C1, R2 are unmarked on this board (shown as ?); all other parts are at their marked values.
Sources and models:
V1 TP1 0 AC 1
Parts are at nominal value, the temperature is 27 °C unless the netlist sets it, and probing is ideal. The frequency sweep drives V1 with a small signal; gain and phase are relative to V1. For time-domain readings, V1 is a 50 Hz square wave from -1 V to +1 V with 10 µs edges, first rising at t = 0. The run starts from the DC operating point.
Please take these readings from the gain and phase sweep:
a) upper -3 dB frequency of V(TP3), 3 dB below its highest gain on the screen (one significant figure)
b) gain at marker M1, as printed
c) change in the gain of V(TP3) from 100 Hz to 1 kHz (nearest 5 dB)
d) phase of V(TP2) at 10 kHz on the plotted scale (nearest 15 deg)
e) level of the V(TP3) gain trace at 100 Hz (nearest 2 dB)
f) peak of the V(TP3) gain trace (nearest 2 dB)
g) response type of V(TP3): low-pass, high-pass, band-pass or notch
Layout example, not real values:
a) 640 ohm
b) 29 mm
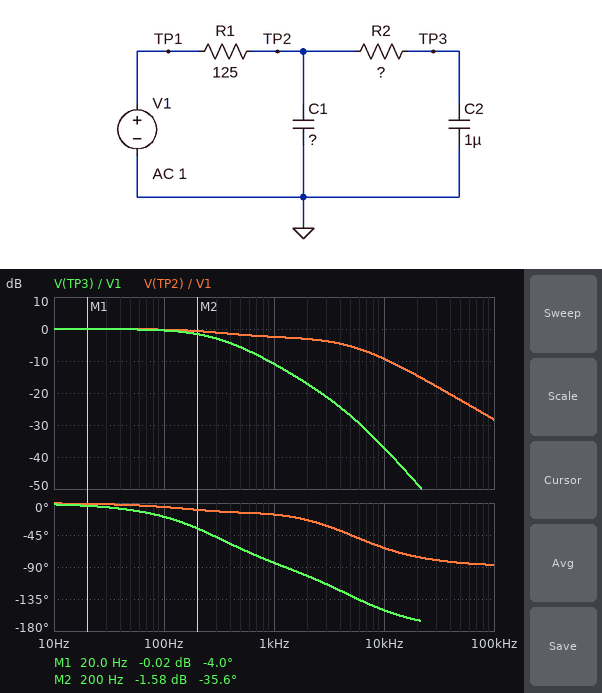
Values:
a) 300 Hz
b) -0.02 dB
c) -10 dB
d) -60 deg
e) 0 dB
f) 0 dB
g) low-pass
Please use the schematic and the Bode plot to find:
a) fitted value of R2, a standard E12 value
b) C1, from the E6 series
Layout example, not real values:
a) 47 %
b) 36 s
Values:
a) 390 Ω
b) 330 nF
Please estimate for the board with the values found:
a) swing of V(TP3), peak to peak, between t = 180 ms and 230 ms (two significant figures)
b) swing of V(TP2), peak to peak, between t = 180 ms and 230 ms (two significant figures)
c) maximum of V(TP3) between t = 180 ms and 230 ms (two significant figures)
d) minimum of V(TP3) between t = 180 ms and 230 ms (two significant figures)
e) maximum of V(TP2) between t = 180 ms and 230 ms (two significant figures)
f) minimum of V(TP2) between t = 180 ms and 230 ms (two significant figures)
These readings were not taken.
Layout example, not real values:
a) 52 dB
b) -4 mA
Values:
a) 2.0 V
b) 2.0 V
c) 1.0 V
d) -1.0 V
e) 1.0 V
f) -1.0 V
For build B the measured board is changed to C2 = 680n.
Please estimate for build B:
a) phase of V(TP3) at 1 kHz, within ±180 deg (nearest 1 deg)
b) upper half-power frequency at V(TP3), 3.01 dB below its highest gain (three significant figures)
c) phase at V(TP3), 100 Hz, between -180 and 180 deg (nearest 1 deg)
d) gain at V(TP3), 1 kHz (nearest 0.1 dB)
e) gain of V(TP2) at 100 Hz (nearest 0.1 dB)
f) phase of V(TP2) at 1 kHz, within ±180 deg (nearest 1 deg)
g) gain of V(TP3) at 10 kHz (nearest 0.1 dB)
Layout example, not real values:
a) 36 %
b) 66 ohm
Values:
a) -77 deg
b) 438 Hz
c) -14 deg
d) -8.0 dB
e) -0.1 dB
f) -18 deg
g) -33.8 dB
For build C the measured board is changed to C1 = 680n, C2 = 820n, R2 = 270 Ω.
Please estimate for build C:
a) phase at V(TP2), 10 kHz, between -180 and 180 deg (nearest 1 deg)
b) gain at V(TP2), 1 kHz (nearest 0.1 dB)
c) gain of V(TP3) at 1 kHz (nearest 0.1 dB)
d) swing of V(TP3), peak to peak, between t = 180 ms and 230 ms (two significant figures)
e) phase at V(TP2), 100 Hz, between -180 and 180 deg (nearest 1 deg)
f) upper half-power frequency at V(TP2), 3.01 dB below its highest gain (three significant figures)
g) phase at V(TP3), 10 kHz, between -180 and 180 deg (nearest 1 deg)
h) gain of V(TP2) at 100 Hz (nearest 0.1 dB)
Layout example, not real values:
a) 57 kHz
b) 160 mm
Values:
a) -75 deg
b) -3.6 dB
c) -8.2 dB
d) 2.0 V
e) -7 deg
f) 793 Hz
g) -161 deg
h) -0.1 dB
